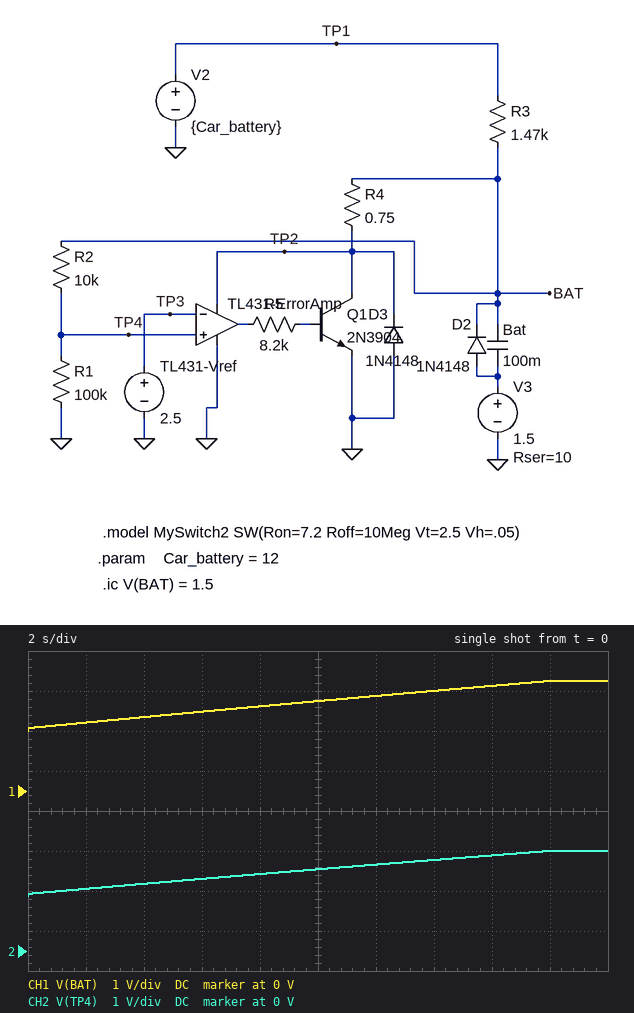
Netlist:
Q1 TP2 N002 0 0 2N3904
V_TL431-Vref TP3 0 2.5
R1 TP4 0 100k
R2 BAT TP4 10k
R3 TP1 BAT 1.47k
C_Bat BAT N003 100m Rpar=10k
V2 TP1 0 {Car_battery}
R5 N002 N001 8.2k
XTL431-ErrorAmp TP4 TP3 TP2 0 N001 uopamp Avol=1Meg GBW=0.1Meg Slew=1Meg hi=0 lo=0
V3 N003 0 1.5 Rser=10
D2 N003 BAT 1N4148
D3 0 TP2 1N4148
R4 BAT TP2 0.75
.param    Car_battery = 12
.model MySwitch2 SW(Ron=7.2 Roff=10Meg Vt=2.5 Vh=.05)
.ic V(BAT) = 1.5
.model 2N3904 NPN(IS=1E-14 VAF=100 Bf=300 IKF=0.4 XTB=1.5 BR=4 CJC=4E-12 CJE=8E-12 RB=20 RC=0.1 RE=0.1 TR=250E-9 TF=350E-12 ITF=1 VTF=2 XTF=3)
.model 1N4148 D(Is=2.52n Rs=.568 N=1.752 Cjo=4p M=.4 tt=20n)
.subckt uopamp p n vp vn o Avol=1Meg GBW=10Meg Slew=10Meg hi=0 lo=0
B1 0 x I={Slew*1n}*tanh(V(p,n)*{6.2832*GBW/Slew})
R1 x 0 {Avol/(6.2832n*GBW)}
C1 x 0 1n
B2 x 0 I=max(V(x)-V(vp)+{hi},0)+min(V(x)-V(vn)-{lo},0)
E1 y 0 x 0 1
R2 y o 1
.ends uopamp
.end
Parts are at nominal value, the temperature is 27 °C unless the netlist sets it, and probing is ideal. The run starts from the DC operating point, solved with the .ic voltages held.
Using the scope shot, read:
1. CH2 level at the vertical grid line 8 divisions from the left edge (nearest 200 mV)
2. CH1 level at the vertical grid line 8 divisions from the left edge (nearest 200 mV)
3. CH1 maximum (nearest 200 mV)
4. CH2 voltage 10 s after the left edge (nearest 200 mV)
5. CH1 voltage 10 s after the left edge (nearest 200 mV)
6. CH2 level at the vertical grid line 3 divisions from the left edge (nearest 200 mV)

2.4 V
2.6 V
2.8 V
2.0 V
2.2 V
1.8 V
